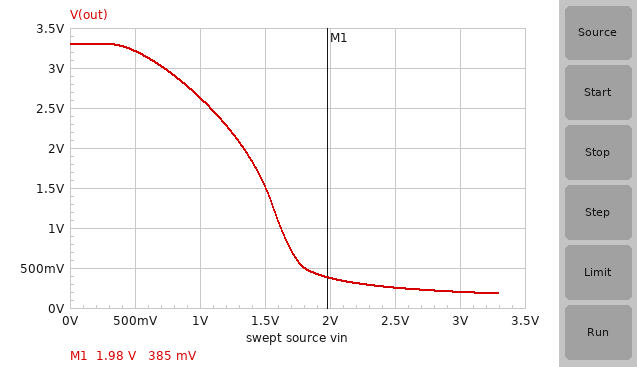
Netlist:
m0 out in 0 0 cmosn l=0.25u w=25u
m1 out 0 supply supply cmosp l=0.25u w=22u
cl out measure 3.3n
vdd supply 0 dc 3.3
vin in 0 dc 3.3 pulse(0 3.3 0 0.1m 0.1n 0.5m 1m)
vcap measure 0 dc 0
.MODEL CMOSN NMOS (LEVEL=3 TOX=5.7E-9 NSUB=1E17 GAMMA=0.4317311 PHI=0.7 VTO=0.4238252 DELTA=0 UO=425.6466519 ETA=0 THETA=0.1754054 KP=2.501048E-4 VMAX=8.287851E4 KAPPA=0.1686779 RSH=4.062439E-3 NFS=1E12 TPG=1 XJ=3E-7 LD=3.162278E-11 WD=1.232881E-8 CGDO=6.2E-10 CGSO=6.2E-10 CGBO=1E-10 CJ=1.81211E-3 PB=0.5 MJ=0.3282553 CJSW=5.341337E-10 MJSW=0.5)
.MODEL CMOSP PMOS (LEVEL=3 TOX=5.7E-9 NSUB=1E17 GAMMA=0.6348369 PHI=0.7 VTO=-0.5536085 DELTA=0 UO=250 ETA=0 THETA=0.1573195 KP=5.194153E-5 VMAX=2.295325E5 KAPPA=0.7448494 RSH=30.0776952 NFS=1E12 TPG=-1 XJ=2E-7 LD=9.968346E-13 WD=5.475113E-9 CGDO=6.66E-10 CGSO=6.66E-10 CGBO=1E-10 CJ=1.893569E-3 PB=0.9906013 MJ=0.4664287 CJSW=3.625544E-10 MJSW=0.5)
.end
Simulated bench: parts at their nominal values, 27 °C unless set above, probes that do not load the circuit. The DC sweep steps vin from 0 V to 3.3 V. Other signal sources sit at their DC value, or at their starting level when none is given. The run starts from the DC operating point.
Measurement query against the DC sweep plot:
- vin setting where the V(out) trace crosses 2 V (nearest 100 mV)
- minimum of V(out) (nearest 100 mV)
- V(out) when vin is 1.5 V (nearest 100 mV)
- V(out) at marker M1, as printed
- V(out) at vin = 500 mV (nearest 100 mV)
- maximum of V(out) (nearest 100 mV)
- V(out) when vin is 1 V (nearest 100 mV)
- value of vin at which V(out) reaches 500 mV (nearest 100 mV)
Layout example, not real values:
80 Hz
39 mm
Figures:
1.3 V
200 mV
1.5 V
385 mV
3.2 V
3.3 V
2.6 V
1.8 V
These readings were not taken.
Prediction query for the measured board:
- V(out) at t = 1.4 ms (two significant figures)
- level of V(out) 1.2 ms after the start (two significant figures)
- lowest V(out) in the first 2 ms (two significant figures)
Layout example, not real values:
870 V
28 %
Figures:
180 mV
180 mV
180 mV
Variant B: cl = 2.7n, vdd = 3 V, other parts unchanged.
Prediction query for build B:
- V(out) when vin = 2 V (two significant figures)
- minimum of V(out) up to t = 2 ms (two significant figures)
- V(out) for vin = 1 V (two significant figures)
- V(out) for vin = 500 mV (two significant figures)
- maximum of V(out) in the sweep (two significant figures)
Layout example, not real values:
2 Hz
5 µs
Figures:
280 mV
150 mV
2.3 V
2.9 V
3.0 V
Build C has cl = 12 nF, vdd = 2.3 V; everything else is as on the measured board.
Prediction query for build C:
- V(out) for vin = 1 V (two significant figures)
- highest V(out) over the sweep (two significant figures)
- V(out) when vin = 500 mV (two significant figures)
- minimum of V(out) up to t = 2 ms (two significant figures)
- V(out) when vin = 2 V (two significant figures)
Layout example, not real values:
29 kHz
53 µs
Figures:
1.4 V
2.3 V
2.2 V
85 mV
140 mV
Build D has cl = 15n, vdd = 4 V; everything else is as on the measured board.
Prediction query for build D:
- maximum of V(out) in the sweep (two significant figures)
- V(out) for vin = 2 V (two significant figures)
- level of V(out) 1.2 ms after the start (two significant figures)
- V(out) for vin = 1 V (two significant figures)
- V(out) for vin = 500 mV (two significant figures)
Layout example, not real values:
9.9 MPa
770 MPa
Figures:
4.0 V
1.1 V
280 mV
3.4 V
3.9 V
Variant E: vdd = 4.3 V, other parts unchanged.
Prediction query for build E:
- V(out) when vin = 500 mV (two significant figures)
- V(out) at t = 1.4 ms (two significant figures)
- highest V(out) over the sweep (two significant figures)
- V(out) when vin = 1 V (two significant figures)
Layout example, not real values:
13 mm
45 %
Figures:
4.2 V
330 mV
4.3 V
3.7 V
